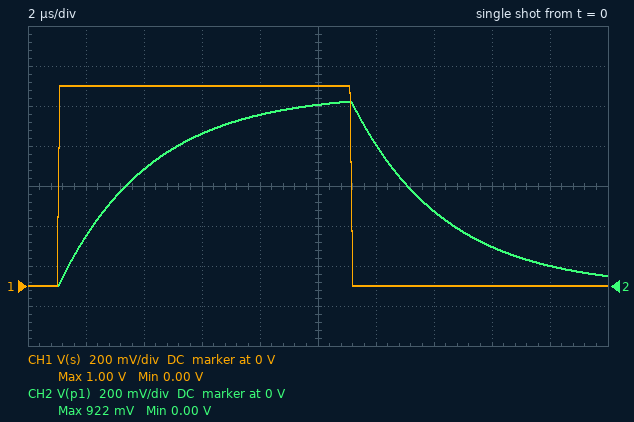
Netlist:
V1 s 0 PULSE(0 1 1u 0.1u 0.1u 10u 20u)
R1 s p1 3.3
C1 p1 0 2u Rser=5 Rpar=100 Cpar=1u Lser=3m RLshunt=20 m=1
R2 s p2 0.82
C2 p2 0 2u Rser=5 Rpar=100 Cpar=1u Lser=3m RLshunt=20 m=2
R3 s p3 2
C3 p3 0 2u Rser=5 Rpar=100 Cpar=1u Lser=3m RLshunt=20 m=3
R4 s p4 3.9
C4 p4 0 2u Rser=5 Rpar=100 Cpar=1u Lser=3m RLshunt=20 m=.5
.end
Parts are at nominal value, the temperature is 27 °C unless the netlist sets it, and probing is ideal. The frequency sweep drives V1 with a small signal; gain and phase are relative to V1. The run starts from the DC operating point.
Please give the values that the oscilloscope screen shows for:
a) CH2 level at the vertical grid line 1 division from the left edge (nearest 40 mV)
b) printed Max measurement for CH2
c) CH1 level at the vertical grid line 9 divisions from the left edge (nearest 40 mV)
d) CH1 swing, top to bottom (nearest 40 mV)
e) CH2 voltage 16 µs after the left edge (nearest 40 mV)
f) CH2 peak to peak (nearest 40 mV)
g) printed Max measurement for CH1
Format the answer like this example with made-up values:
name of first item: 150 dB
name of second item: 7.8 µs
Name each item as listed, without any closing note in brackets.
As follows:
CH2 level at the vertical grid line 1 division from the left edge: 240 mV
printed Max measurement for CH2: 922 mV
CH1 level at the vertical grid line 9 divisions from the left edge: 0 V
CH1 swing, top to bottom: 1.00 V
CH2 voltage 16 µs after the left edge: 200 mV
CH2 peak to peak: 920 mV
printed Max measurement for CH1: 1.00 V
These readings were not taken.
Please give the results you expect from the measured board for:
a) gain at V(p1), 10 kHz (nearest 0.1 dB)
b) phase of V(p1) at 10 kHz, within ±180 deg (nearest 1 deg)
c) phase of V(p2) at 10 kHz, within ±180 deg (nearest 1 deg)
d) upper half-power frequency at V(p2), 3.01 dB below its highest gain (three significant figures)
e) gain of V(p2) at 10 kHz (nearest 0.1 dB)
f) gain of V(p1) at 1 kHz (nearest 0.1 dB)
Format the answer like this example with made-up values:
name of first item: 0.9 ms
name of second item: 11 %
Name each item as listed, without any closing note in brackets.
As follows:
gain at V(p1), 10 kHz: -0.4 dB
phase of V(p1) at 10 kHz, within ±180 deg: -10 deg
phase of V(p2) at 10 kHz, within ±180 deg: -3 deg
upper half-power frequency at V(p2), 3.01 dB below its highest gain: 196 kHz
gain of V(p2) at 10 kHz: -0.1 dB
gain of V(p1) at 1 kHz: -0.3 dB
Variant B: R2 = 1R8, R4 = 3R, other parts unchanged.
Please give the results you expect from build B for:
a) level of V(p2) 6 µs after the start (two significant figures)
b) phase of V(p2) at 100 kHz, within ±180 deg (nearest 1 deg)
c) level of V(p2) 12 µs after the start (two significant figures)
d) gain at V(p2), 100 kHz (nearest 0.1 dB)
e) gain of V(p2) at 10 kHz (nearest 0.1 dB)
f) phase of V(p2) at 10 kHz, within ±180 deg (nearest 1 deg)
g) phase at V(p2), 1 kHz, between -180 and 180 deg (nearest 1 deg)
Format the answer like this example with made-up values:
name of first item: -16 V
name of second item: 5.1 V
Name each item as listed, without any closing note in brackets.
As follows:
level of V(p2) 6 µs after the start: 920 mV
phase of V(p2) at 100 kHz, within ±180 deg: -48 deg
level of V(p2) 12 µs after the start: 600 mV
gain at V(p2), 100 kHz: -3.6 dB
gain of V(p2) at 10 kHz: -0.2 dB
phase of V(p2) at 10 kHz, within ±180 deg: -6 deg
phase at V(p2), 1 kHz, between -180 and 180 deg: -5 deg
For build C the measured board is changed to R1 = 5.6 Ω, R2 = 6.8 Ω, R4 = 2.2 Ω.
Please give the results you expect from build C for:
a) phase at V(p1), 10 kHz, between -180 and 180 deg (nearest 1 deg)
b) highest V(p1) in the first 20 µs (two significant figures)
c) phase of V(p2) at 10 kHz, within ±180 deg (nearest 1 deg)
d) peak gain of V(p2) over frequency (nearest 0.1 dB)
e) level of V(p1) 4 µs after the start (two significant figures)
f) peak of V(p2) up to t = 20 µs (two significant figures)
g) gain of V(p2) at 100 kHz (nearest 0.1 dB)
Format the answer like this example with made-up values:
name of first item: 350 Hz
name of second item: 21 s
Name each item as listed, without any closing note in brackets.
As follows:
phase at V(p1), 10 kHz, between -180 and 180 deg: -17 deg
highest V(p1) in the first 20 µs: 800 mV
phase of V(p2) at 10 kHz, within ±180 deg: -20 deg
peak gain of V(p2) over frequency: -0.6 dB
level of V(p1) 4 µs after the start: 400 mV
peak of V(p2) up to t = 20 µs: 740 mV
gain of V(p2) at 100 kHz: -12.9 dB
